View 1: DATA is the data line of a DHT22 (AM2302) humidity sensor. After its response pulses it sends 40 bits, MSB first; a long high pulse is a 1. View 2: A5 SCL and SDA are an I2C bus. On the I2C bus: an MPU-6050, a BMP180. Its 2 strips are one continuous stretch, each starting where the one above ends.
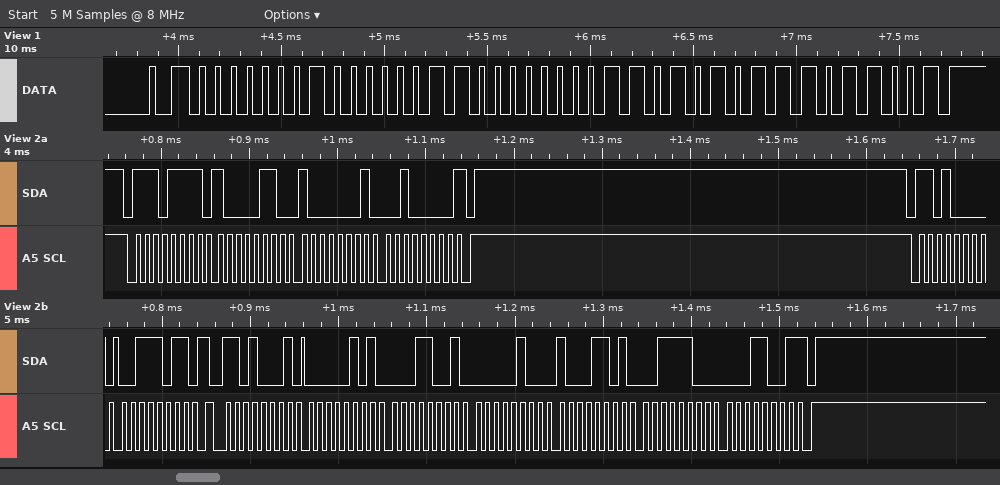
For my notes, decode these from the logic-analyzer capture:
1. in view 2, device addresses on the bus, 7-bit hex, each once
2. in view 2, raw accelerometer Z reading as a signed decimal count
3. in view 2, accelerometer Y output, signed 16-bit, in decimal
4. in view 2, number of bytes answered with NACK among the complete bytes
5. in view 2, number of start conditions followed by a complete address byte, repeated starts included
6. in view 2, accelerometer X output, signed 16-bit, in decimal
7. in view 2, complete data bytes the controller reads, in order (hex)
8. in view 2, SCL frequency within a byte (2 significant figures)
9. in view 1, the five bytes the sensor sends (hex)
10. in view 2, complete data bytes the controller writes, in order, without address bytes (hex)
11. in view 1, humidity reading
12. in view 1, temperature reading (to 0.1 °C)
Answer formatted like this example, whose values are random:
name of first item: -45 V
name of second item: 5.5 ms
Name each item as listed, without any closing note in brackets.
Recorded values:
in view 2, device addresses on the bus, 7-bit hex, each once: 0x77 0x68
in view 2, raw accelerometer Z reading as a signed decimal count: 15385
in view 2, accelerometer Y output, signed 16-bit, in decimal: 1165
in view 2, number of bytes answered with NACK among the complete bytes: 2
in view 2, number of start conditions followed by a complete address byte, repeated starts included: 3
in view 2, accelerometer X output, signed 16-bit, in decimal: 1305
in view 2, complete data bytes the controller reads, in order: 86 81 20 05 19 04 8D 3C 19
in view 2, SCL frequency within a byte: 100 kHz
in view 1, the five bytes the sensor sends: 01 03 00 D5 D9
in view 2, complete data bytes the controller writes, in order, without address bytes: 3B
in view 1, humidity reading: 25.9 %
in view 1, temperature reading: 21.3 °C
